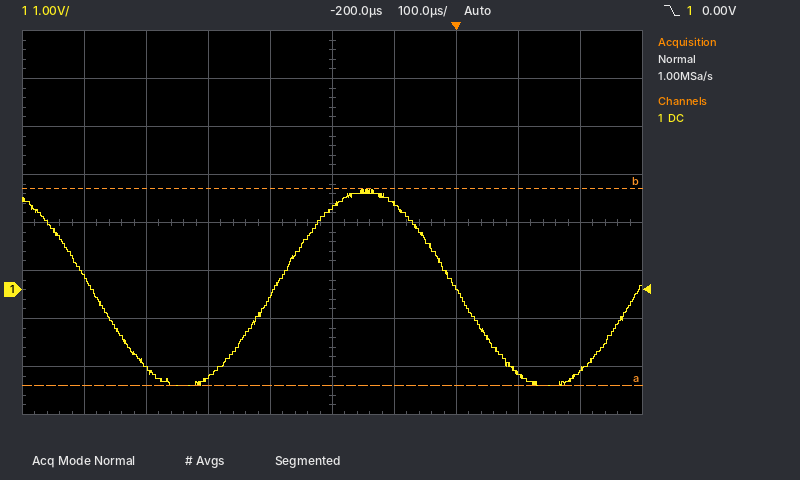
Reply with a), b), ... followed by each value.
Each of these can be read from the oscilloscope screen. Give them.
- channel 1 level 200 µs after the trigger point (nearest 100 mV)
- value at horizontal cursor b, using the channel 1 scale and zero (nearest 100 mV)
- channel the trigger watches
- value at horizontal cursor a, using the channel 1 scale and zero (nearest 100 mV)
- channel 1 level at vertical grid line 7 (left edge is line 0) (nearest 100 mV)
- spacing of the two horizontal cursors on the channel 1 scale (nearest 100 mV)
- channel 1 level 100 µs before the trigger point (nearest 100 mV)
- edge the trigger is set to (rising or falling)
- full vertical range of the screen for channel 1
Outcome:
a) -1.7 V
b) 2.1 V
c) channel 1
d) -2.0 V
e) 0.0 V
f) 4.1 V
g) 1.8 V
h) falling
i) 8 V
